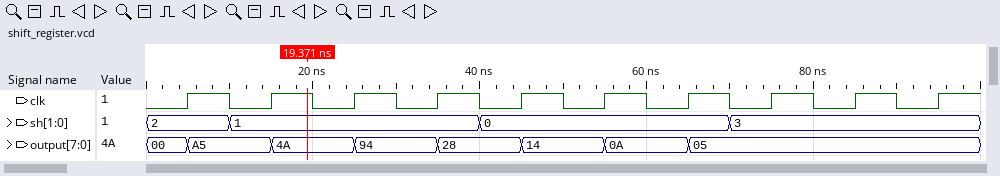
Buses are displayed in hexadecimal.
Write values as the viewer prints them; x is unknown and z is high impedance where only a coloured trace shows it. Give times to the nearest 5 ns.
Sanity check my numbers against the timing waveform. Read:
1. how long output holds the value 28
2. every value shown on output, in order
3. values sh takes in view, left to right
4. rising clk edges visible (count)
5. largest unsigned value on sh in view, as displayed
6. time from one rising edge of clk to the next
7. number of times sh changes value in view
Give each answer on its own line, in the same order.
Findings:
10 ns
00, A5, 4A, 94, 28, 14, 0A, 05
2, 1, 0, 3
10
3
10 ns
3
